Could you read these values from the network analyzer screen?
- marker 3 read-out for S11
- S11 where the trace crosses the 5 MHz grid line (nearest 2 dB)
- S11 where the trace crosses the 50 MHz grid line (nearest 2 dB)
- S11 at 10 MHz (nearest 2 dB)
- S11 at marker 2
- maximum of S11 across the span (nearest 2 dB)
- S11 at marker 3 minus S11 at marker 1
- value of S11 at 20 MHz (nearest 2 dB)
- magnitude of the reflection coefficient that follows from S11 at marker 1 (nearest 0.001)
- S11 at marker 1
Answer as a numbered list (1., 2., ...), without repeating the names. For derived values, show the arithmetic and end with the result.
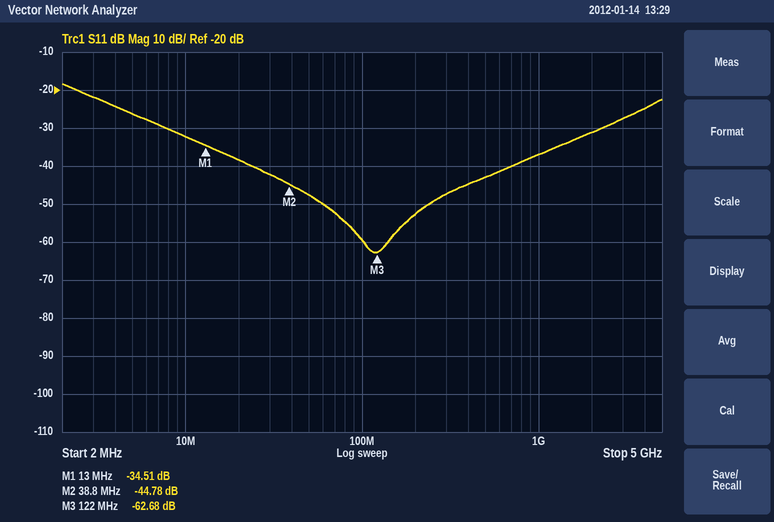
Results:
1. -62.68 dB
2. -26 dB
3. -48 dB
4. -32 dB
5. -44.78 dB
6. -18 dB
7. -62.68 − (-34.51) = -28.17 dB
8. -38 dB
9. 10^(-34.51/20) ≈ 0.019
10. -34.51 dB
